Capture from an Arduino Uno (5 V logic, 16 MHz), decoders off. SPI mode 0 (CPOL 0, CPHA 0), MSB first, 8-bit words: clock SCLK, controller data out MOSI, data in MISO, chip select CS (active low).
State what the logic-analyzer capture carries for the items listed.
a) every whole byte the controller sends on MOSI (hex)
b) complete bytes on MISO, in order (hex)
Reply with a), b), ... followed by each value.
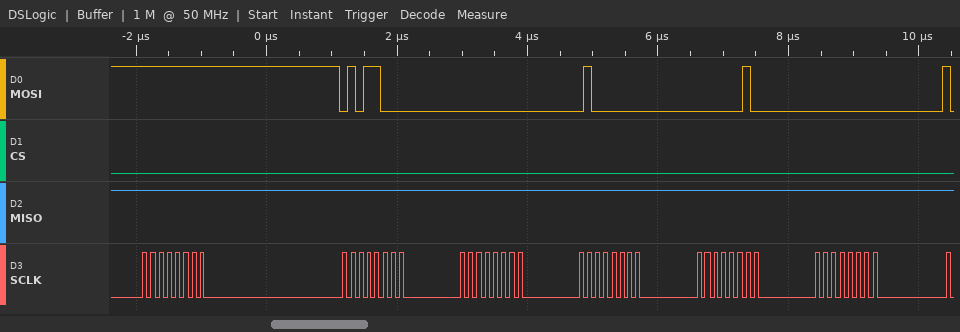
a) FF 58 00 40 02 00
b) FF FF FF FF FF FF
